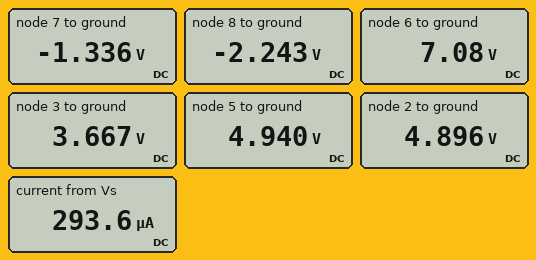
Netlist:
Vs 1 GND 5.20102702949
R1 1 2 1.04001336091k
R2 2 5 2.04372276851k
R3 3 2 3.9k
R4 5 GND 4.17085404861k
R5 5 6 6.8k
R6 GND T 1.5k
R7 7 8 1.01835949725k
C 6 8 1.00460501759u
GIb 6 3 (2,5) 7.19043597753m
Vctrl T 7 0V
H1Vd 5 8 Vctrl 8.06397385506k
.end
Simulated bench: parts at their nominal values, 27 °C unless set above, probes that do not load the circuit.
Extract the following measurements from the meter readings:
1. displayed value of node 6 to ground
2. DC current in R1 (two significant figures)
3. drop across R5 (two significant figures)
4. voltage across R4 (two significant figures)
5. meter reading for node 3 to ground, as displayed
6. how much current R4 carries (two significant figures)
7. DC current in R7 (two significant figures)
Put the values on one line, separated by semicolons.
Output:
7.08 V; 290 µA; 2.1 V; 4.9 V; 3.667 V; 1.2 mA; 890 µA
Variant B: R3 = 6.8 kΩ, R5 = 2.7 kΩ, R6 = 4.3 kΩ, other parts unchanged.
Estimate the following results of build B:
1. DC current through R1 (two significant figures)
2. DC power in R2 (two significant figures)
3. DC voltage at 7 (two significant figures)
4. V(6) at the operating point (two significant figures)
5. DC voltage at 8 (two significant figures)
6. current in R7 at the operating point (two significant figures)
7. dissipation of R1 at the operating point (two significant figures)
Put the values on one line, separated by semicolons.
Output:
730 µA; 5.8 µW; -9.2 V; 3.7 V; -11 V; 2.1 mA; 550 µW
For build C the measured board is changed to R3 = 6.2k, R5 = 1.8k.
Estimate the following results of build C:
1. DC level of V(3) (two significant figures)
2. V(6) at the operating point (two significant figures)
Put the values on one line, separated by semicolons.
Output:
2.9 V; 5.5 V
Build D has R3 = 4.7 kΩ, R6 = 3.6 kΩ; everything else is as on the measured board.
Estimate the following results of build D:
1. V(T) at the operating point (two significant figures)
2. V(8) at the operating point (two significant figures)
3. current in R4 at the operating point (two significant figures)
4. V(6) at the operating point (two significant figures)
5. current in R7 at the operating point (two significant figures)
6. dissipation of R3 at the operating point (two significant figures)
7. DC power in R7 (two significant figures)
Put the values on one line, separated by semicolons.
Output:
-5.7 V; -7.3 V; 1.3 mA; 3.4 V; 1.6 mA; 410 µW; 2.5 mW
